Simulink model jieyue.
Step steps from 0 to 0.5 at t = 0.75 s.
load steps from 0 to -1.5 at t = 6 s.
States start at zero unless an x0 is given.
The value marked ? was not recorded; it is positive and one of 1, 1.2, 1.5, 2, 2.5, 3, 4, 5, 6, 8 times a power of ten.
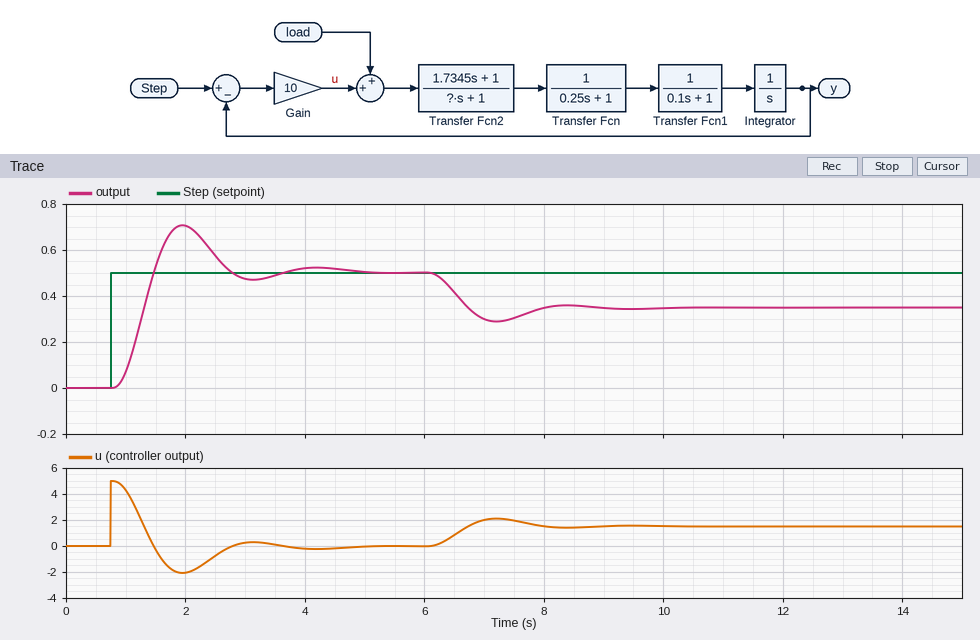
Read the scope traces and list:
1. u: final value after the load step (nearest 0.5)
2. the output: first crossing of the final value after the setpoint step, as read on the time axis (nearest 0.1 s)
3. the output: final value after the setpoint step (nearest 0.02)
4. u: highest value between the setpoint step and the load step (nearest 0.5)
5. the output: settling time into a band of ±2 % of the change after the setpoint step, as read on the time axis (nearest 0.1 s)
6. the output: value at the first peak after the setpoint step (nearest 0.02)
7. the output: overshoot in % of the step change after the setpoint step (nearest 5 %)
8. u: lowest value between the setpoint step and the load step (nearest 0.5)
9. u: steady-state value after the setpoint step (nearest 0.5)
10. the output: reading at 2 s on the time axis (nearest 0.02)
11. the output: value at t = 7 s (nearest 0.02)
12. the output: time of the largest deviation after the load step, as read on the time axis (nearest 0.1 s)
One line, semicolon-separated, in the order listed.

1.5; 1.5 s; 0.50; 5.0; 4.8 s; 0.70; 40 %; -2.0; 0.0; 0.70; 0.30; 7.2 s
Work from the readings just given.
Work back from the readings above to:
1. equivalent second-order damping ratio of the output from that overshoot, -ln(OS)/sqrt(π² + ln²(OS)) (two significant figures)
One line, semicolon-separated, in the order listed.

0.28
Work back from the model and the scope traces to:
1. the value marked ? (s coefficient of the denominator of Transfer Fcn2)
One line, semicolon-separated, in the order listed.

6
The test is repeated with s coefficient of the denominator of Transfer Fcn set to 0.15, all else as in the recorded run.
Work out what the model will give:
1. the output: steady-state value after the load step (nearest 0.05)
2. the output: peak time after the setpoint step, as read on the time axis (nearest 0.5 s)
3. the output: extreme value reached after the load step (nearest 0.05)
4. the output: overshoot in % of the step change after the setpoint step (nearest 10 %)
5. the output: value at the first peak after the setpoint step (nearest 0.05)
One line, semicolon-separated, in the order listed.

0.35; 2.0 s; 0.30; 30 %; 0.65
